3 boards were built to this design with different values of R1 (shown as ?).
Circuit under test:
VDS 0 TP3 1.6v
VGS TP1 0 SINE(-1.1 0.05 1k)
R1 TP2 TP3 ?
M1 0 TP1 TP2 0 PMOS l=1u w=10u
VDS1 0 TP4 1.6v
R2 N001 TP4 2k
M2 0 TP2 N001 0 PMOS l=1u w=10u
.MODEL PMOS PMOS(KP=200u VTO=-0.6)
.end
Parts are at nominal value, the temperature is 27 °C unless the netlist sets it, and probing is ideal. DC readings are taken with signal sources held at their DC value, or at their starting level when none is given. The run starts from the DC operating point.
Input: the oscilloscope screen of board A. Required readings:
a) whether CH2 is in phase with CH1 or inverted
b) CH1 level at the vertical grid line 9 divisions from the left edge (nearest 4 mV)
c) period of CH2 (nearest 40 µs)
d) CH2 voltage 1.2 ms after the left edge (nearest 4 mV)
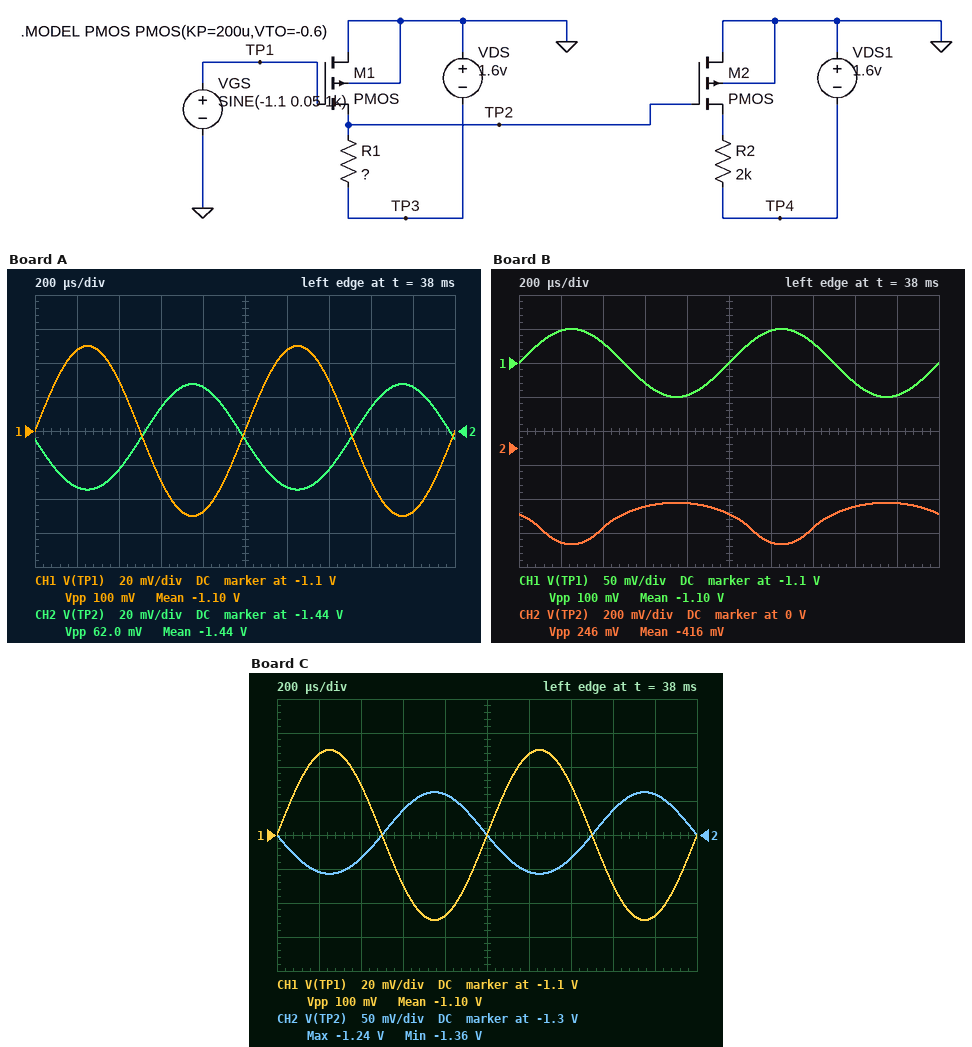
inverted
-1.148 V
1.00 ms
-1.472 V
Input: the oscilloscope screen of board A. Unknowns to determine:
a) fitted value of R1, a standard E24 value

620 Ω
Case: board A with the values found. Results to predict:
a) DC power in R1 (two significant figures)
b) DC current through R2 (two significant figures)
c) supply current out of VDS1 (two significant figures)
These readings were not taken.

39 µW
570 µA
570 µA
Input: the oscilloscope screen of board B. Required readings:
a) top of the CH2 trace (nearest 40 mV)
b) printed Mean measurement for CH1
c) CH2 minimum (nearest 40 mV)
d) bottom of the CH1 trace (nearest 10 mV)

-320 mV
-1.10 V
-560 mV
-1.15 V
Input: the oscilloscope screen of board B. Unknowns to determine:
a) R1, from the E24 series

5.1 kΩ
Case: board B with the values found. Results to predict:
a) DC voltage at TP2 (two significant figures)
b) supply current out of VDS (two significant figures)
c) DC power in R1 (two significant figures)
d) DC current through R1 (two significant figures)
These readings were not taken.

-390 mV
240 µA
290 µW
240 µA
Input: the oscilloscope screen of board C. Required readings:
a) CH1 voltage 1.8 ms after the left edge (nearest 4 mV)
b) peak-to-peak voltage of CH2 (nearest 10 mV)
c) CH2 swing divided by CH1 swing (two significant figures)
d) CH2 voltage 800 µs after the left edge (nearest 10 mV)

-1.148 V
120 mV
1.2
-1.24 V
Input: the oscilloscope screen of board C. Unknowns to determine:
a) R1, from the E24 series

1.2 kΩ
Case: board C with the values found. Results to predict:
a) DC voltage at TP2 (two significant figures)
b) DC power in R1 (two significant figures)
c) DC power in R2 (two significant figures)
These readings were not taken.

-1.3 V
75 µW
470 µW
